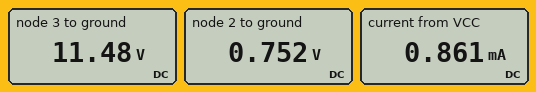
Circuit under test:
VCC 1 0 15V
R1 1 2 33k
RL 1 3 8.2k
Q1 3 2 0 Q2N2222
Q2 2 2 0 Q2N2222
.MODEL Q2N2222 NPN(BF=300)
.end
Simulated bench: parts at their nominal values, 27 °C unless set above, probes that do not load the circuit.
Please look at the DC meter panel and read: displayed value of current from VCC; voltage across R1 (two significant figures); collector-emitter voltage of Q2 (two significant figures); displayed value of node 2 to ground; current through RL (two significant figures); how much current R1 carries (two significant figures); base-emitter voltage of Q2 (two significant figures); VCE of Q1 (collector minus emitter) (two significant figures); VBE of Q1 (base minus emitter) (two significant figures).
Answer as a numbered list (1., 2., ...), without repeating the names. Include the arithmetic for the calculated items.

1. 0.861 mA
2. 15 V - 752 mV = 14 V
3. 752 mV = 750 mV
4. 0.752 V
5. (15 V - 11.48 V) / 8.2 kΩ = 430 µA
6. (15 V - 752 mV) / 33 kΩ = 430 µA
7. 752 mV = 750 mV
8. 11.48 V = 11 V
9. 752 mV = 750 mV
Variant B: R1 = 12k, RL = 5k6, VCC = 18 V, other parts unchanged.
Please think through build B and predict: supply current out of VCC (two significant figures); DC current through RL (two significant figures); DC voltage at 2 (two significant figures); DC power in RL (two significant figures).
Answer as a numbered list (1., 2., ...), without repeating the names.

1. 2.9 mA
2. 1.4 mA
3. 780 mV
4. 11 mW
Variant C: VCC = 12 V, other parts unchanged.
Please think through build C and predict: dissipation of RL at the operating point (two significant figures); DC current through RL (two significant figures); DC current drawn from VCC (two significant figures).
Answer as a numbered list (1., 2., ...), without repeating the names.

1. 940 µW
2. 340 µA
3. 680 µA
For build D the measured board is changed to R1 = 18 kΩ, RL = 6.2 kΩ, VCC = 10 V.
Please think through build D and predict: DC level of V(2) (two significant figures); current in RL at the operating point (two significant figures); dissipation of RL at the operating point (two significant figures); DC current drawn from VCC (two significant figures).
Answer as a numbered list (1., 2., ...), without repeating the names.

1. 760 mV
2. 510 µA
3. 1.6 mW
4. 1.0 mA
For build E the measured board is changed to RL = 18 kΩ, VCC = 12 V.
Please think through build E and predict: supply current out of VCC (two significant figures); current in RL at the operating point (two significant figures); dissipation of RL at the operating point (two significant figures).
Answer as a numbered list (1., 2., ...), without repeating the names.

1. 680 µA
2. 340 µA
3. 2.1 mW
